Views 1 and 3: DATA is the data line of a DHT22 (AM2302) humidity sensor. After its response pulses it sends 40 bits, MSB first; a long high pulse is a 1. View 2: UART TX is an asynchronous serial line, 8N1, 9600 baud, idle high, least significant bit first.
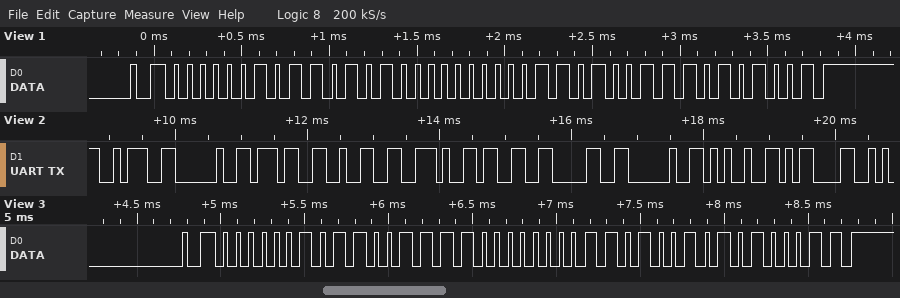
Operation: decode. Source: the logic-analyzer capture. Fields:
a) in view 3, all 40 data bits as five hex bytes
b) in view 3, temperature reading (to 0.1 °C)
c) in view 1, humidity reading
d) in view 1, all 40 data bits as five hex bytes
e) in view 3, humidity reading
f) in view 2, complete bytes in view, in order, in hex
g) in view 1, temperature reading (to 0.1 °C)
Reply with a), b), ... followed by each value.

a) 02 CF 00 D2 A3
b) 21.0 °C
c) 72.4 %
d) 02 D4 00 D3 A9
e) 71.9 %
f) 3A 20 37 32 2E 33 30 20 25 0D
g) 21.1 °C
